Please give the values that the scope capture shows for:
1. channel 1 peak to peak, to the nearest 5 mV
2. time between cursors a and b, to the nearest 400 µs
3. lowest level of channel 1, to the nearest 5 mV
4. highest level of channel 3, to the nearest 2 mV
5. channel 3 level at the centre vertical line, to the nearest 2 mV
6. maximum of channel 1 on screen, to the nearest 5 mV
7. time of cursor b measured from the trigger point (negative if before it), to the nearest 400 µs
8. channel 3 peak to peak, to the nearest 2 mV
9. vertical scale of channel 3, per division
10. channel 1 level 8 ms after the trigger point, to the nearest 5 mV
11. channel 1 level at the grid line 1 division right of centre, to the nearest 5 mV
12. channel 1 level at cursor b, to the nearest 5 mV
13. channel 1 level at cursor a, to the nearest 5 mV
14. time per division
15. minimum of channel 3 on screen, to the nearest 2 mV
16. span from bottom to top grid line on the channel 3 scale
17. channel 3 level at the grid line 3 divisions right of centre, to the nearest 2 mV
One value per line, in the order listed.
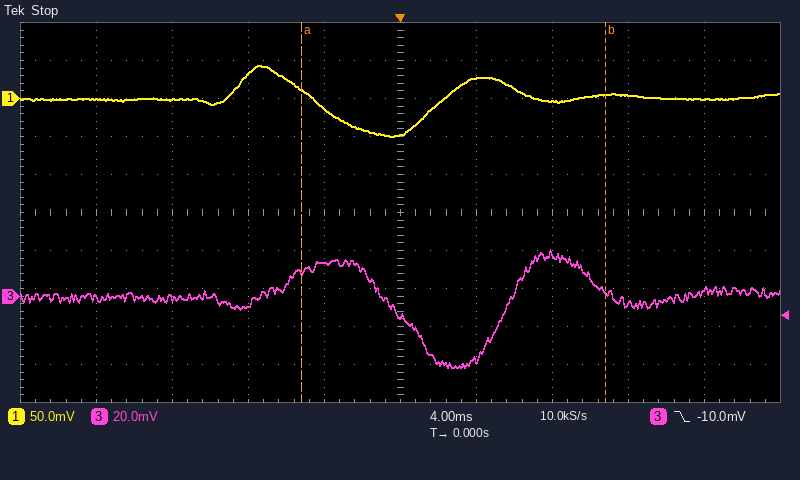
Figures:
95 mV
16.0 ms
-50 mV
24 mV
-10 mV
45 mV
+10.8 ms
62 mV
20 mV
-5 mV
25 mV
5 mV
10 mV
4 ms
-38 mV
200 mV
-4 mV
